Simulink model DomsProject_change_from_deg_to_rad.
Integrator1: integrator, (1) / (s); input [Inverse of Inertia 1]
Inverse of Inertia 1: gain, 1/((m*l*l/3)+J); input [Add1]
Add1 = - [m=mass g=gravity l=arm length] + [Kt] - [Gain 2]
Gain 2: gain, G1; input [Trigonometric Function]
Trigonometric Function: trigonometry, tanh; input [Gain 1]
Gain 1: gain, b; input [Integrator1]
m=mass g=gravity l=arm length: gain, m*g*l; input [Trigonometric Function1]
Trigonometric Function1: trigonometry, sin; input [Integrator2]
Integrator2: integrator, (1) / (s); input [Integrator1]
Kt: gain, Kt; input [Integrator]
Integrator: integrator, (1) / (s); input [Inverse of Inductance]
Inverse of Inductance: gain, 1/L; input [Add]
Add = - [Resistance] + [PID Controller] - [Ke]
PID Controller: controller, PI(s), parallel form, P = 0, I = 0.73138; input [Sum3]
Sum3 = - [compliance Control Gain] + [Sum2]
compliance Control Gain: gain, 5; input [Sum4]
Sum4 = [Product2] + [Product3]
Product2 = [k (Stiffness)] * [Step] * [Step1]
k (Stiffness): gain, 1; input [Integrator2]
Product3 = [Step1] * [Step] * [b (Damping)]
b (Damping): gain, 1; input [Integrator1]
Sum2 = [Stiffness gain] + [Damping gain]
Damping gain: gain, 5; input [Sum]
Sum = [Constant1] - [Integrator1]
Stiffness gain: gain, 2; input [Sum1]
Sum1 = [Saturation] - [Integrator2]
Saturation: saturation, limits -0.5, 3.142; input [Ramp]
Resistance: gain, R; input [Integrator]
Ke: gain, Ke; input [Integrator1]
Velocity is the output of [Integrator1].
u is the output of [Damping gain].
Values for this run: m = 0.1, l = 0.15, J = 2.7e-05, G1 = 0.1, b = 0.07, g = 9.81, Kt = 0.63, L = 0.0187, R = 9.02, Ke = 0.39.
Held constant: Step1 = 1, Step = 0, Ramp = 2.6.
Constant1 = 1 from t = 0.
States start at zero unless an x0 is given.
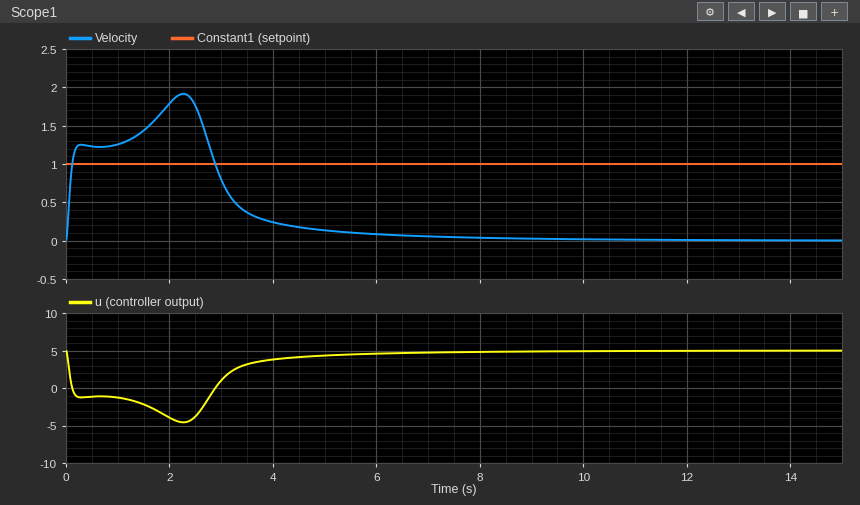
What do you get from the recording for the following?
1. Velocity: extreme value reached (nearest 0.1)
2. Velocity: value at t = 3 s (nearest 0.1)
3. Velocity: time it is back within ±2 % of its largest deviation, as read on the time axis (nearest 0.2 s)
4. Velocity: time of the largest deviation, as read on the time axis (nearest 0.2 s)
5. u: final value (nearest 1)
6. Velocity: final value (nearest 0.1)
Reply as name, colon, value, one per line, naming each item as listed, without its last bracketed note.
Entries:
Velocity: extreme value reached: 1.9
Velocity: value at t = 3 s: 0.8
Velocity: time it is back within ±2 % of its largest deviation, as read on the time axis: 8.0 s
Velocity: time of the largest deviation, as read on the time axis: 2.2 s
u: final value: 5
Velocity: final value: 0.0
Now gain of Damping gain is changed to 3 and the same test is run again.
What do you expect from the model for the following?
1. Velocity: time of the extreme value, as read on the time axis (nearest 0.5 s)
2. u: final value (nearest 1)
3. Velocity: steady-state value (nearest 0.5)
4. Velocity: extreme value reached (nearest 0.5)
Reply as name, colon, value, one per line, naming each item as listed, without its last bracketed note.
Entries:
Velocity: time of the extreme value, as read on the time axis: 2.0 s
u: final value: 3
Velocity: steady-state value: 0.0
Velocity: extreme value reached: 3.0
